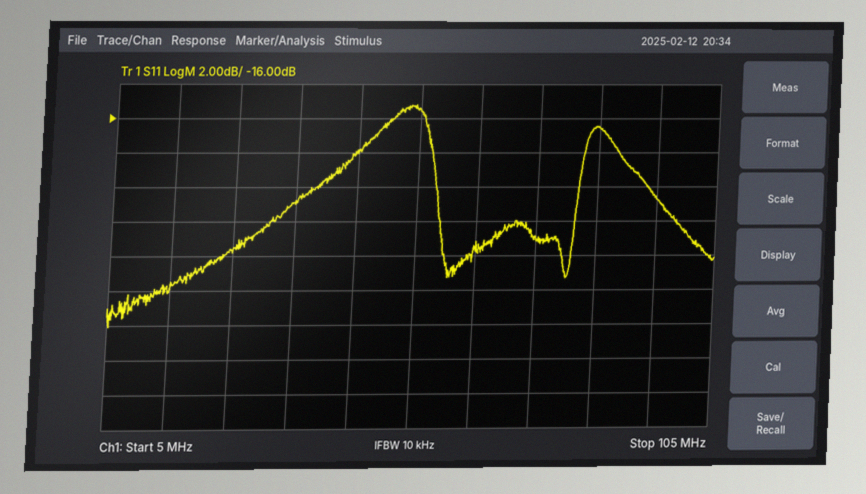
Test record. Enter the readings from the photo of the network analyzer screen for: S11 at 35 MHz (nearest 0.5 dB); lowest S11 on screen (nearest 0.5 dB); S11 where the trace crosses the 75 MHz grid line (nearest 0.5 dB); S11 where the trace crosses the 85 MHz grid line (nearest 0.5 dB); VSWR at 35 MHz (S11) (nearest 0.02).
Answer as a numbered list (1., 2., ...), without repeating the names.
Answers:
1. -21.0 dB
2. -28.0 dB
3. -23.0 dB
4. -16.5 dB
5. 1.20
